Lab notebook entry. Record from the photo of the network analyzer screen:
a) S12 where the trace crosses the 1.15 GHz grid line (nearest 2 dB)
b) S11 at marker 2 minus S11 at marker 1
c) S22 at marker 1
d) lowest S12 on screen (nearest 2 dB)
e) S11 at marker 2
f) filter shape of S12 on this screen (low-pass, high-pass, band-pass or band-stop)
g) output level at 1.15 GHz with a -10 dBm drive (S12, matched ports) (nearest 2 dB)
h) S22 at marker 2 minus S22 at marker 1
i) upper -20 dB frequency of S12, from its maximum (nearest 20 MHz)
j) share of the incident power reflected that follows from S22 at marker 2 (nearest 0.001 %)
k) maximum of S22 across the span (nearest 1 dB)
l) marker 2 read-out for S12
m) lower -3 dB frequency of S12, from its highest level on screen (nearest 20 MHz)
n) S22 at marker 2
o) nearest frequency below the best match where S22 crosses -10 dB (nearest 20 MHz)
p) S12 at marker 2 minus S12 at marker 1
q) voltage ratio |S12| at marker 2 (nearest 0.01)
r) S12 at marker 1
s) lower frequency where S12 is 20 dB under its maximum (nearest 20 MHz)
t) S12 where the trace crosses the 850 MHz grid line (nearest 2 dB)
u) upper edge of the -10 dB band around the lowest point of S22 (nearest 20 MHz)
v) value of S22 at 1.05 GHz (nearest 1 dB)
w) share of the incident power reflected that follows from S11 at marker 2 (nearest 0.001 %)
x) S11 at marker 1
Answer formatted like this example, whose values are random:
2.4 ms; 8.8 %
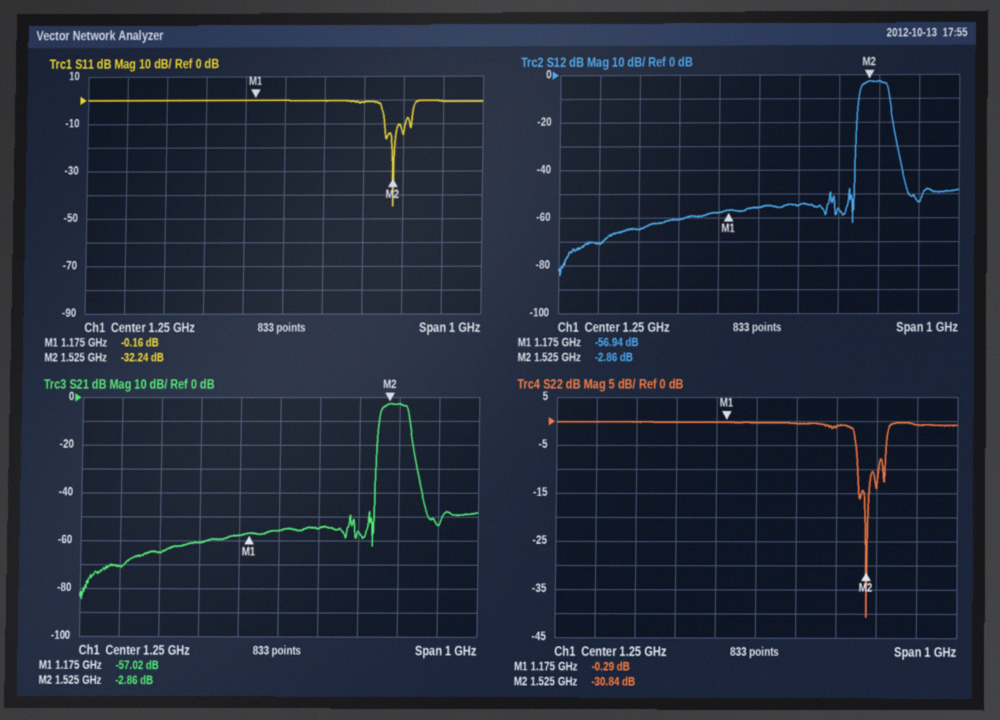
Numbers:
-58 dB; -32.08 dB; -0.29 dB; -84 dB; -32.24 dB; band-pass; -68 dBm; -30.55 dB; 1.58 GHz; 0.082 %; 0 dB; -2.86 dB; 1.50 GHz; -30.84 dB; 1.50 GHz; 54.08 dB; 0.72; -56.94 dB; 1.50 GHz; -70 dB; 1.56 GHz; 0 dB; 0.060 %; -0.16 dB
